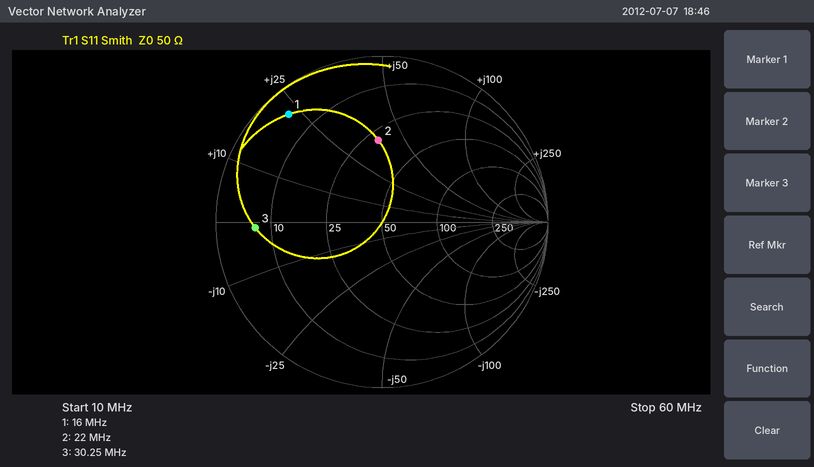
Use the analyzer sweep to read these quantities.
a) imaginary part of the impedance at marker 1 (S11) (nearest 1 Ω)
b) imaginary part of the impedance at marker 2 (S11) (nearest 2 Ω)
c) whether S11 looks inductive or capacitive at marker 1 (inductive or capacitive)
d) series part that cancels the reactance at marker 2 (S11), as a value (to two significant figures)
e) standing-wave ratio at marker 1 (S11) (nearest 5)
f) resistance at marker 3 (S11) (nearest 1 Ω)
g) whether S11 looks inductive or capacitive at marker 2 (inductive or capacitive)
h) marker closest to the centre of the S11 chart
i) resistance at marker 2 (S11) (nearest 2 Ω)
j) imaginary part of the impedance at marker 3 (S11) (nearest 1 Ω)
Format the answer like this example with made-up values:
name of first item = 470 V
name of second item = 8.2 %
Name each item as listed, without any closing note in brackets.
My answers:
imaginary part of the impedance at marker 1 (S11) = +23 Ω
imaginary part of the impedance at marker 2 (S11) = +38 Ω
whether S11 looks inductive or capacitive at marker 1 = inductive
series part that cancels the reactance at marker 2 (S11), as a value = 190 pF
standing-wave ratio at marker 1 (S11) = 15
resistance at marker 3 (S11) = 7 Ω
whether S11 looks inductive or capacitive at marker 2 = inductive
marker closest to the centre of the S11 chart = marker 2
resistance at marker 2 (S11) = 30 Ω
imaginary part of the impedance at marker 3 (S11) = -1 Ω
